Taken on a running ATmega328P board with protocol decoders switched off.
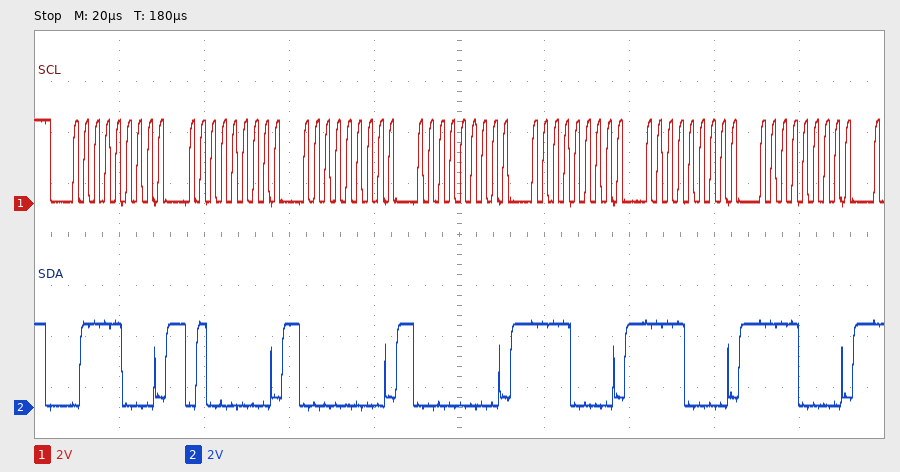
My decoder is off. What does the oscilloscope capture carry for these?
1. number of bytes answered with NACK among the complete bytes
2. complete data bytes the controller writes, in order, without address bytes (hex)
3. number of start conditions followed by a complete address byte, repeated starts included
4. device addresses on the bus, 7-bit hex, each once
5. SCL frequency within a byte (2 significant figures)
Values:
0
40 00 00 F0 F0 F0
1
0x3C
400 kHz
